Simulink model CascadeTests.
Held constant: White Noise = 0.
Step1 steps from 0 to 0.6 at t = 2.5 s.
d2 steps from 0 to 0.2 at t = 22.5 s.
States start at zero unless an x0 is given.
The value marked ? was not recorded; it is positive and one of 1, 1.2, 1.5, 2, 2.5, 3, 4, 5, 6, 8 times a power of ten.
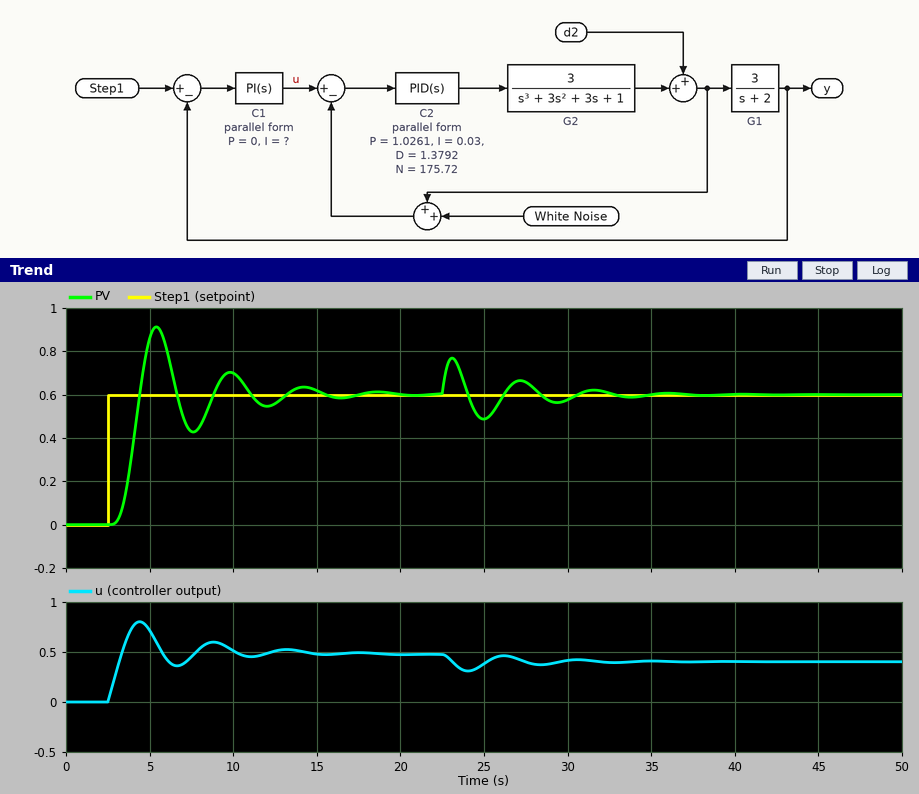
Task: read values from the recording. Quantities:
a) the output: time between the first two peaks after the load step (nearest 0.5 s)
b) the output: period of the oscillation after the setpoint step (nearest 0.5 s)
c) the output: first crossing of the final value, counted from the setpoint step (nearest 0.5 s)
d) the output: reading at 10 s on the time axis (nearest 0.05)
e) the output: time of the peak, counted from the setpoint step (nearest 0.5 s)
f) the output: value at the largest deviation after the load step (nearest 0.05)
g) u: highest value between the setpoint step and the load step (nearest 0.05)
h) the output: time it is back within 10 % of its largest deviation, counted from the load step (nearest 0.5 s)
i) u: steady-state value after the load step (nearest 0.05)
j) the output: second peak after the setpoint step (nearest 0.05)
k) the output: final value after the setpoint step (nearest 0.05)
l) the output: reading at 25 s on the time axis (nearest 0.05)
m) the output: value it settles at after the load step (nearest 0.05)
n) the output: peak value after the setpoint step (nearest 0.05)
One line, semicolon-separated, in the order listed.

4.0 s; 4.5 s; 2.0 s; 0.70; 3.0 s; 0.75; 0.80; 9.5 s; 0.40; 0.70; 0.60; 0.50; 0.60; 0.90
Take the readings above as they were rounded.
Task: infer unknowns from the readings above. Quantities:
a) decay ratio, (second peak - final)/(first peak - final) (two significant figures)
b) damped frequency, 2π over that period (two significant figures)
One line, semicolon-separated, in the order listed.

0.33; 1.4 rad/s
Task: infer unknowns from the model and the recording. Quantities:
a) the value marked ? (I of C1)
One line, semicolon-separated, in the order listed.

1
